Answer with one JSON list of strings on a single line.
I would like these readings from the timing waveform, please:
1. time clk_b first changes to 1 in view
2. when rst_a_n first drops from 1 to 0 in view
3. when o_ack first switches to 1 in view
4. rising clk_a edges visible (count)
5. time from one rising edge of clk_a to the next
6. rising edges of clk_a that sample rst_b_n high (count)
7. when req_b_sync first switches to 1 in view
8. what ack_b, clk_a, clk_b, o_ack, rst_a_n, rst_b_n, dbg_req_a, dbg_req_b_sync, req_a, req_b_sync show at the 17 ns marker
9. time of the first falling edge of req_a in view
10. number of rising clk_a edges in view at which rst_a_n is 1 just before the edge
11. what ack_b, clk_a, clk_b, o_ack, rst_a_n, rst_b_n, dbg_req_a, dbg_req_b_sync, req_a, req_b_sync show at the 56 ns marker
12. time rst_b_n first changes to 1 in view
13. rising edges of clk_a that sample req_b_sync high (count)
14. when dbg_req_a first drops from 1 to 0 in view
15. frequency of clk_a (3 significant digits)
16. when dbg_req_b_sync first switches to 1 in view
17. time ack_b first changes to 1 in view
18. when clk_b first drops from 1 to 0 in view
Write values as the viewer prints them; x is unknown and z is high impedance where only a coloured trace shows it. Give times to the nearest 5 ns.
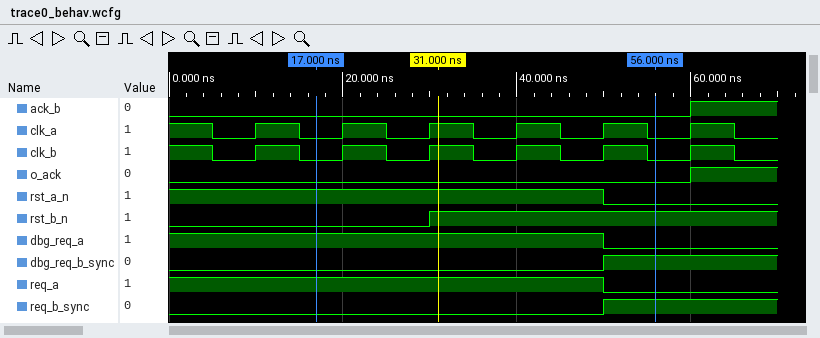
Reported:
["10 ns", "50 ns", "60 ns", "6", "10 ns", "3", "50 ns", "ack_b=0, clk_a=0, clk_b=0, o_ack=0, rst_a_n=1, rst_b_n=0, dbg_req_a=1, dbg_req_b_sync=0, req_a=1, req_b_sync=0", "50 ns", "5", "ack_b=0, clk_a=0, clk_b=0, o_ack=0, rst_a_n=0, rst_b_n=1, dbg_req_a=0, dbg_req_b_sync=1, req_a=0, req_b_sync=1", "30 ns", "1", "50 ns", "100 MHz", "50 ns", "60 ns", "5 ns"]
